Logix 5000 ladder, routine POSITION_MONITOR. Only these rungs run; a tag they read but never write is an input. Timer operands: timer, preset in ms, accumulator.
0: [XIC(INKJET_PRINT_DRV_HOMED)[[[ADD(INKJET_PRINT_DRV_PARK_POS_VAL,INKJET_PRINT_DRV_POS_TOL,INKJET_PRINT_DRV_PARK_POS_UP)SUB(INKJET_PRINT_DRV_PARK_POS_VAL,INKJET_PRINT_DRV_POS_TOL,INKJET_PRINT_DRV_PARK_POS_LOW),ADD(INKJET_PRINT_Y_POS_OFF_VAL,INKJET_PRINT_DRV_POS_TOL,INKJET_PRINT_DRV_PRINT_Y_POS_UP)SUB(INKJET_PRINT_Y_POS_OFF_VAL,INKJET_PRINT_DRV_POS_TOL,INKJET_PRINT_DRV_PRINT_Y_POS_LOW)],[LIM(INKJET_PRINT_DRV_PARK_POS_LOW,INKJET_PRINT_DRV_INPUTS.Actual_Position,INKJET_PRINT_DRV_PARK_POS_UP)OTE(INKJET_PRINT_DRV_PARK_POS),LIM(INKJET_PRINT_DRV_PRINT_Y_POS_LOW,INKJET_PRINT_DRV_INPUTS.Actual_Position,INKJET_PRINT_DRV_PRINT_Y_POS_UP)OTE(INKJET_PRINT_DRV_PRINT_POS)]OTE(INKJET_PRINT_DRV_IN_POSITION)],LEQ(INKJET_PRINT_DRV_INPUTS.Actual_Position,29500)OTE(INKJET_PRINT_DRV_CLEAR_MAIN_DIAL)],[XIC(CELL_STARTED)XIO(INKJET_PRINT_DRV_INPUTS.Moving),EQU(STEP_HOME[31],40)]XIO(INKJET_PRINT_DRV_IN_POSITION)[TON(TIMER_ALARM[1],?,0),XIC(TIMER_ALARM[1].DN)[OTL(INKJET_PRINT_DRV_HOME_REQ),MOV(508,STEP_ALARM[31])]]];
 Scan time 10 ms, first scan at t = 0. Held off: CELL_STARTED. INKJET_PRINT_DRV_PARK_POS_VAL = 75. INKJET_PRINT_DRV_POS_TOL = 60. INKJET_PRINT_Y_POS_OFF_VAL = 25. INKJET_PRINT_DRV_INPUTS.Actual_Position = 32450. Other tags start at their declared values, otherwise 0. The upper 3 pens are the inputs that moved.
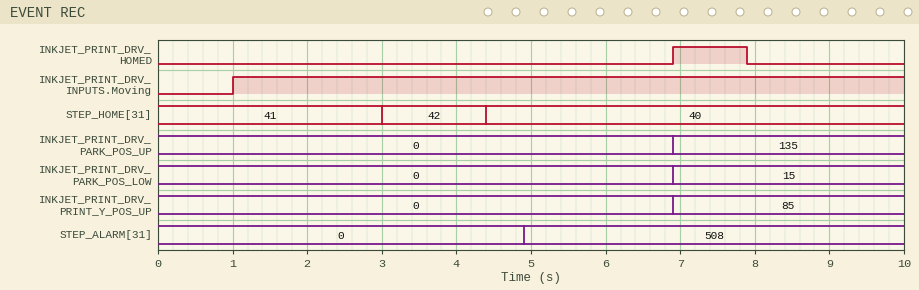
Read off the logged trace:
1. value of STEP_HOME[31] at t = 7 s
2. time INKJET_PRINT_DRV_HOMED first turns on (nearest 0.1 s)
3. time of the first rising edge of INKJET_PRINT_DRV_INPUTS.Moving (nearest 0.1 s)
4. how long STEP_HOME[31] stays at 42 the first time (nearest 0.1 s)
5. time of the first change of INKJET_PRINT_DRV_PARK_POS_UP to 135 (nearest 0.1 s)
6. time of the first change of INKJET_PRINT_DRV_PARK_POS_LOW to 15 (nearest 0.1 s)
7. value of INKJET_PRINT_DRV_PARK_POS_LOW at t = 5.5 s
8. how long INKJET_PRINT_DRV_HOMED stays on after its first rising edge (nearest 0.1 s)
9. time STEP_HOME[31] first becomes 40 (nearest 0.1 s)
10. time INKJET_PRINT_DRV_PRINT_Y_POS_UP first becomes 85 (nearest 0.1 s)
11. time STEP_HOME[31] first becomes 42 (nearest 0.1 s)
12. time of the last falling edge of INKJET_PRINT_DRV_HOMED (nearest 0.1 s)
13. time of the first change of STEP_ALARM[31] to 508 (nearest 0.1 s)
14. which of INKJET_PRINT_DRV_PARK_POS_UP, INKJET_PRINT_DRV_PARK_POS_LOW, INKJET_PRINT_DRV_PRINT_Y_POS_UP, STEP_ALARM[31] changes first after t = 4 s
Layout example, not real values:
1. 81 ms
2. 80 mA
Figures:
1. 40
2. 6.9 s
3. 1.0 s
4. 1.4 s
5. 6.9 s
6. 6.9 s
7. 0
8. 1.0 s
9. 4.4 s
10. 6.9 s
11. 3.0 s
12. 7.9 s
13. 4.9 s
14. STEP_ALARM[31]
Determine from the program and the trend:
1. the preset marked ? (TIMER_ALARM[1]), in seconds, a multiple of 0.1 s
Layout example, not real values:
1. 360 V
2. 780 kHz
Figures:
1. 0.5 s
